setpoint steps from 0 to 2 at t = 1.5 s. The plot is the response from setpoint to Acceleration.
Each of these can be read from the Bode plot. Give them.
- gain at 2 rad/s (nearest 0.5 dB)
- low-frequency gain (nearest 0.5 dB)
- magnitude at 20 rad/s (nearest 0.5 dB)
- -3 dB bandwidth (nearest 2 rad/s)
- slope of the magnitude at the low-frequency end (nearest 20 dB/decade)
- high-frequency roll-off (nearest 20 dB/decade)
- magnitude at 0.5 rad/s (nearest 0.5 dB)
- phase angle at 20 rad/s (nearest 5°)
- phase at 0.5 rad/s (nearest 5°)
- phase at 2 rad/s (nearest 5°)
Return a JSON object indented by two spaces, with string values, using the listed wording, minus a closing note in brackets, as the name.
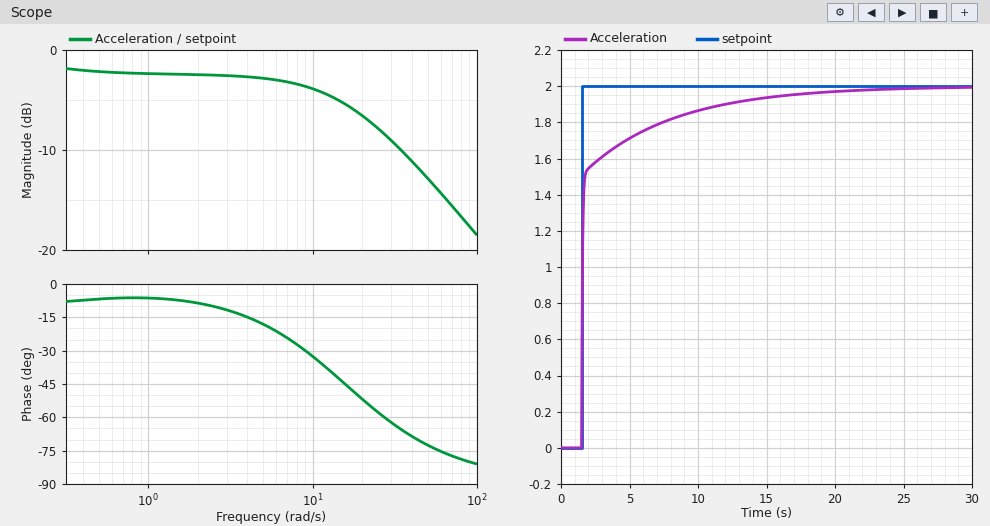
{
  "gain at 2 rad/s": "-2.5 dB",
  "low-frequency gain": "-2.0 dB",
  "magnitude at 20 rad/s": "-6.5 dB",
  "-3 dB bandwidth": "14 rad/s",
  "slope of the magnitude at the low-frequency end": "0 dB/decade",
  "high-frequency roll-off": "-20 dB/decade",
  "magnitude at 0.5 rad/s": "-2.0 dB",
  "phase angle at 20 rad/s": "-50°",
  "phase at 0.5 rad/s": "-5°",
  "phase at 2 rad/s": "-10°"
}
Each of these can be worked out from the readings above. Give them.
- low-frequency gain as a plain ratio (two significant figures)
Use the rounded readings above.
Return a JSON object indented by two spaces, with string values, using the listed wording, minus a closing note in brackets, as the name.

{
  "low-frequency gain as a plain ratio": "0.79"
}
